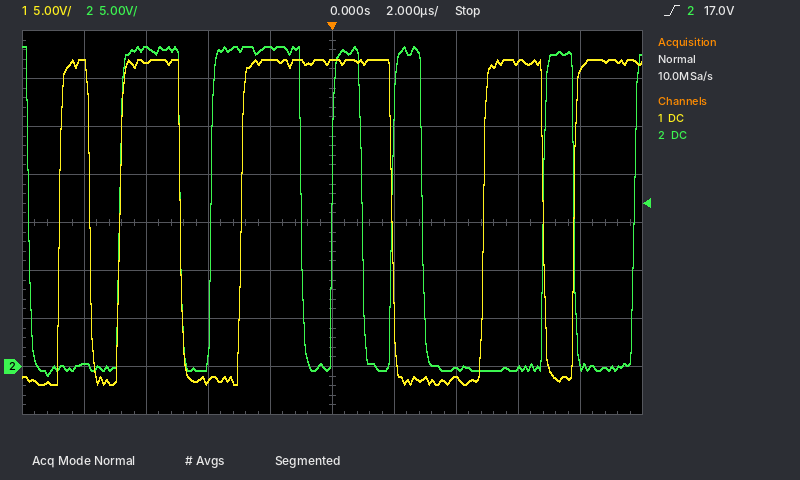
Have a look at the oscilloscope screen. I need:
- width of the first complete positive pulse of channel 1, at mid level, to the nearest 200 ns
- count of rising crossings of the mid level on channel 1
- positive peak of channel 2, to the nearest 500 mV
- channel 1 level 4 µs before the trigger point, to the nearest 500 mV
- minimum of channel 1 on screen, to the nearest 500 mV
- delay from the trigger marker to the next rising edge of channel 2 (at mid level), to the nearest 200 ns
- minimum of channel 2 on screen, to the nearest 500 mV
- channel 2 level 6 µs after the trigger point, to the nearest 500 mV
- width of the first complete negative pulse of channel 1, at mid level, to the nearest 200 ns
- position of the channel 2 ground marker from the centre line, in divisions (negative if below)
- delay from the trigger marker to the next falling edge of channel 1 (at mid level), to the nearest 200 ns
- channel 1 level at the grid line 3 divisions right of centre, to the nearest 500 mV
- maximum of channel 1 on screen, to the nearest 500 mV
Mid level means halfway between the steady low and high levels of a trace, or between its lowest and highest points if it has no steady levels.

1.0 µs
5
33.5 V
-1.5 V
-2.0 V
2.0 µs
-1.0 V
0.0 V
1.0 µs
-3.0 div
2.0 µs
31.5 V
32.0 V
